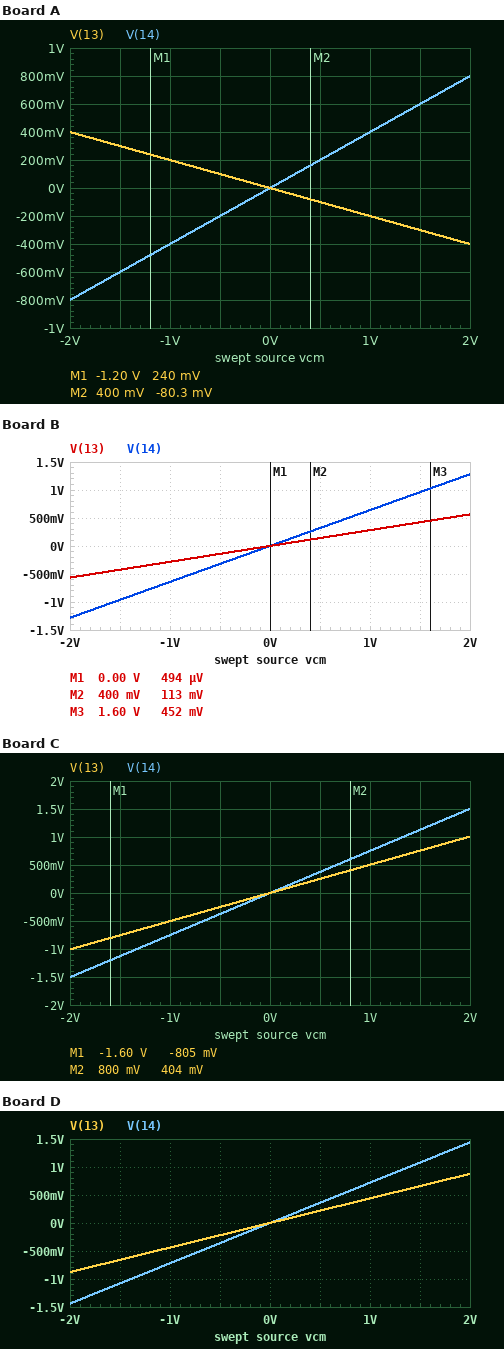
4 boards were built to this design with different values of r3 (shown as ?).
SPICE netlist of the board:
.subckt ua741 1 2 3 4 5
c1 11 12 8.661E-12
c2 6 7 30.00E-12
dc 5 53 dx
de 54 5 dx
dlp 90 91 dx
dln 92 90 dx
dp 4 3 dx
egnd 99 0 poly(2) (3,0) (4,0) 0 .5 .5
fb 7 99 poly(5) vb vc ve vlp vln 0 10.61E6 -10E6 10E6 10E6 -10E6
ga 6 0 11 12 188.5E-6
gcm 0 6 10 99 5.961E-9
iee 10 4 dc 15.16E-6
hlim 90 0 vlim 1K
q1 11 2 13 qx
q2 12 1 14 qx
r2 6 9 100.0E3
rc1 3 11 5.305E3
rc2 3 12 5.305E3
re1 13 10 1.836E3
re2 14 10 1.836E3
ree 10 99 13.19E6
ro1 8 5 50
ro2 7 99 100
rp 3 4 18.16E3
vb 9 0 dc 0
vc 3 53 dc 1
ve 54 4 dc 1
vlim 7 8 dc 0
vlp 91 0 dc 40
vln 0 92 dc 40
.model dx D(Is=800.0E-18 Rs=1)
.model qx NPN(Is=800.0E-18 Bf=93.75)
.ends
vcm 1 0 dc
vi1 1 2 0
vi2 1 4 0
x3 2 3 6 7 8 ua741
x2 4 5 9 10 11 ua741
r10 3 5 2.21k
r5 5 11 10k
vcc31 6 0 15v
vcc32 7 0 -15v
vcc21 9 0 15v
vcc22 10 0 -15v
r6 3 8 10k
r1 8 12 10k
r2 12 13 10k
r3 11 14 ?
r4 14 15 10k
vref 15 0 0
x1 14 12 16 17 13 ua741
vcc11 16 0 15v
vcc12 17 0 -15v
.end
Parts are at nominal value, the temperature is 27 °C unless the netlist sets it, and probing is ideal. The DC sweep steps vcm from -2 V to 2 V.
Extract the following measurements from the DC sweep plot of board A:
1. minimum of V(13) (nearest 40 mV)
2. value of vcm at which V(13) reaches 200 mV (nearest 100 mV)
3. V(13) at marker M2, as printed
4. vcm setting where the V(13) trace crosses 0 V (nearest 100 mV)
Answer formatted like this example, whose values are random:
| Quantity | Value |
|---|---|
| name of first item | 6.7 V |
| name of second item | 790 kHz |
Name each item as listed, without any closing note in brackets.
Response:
| Quantity | Value |
|---|---|
| minimum of V(13) | -400 mV |
| value of vcm at which V(13) reaches 200 mV | -1.0 V |
| V(13) at marker M2, as printed | -80.3 mV |
| vcm setting where the V(13) trace crosses 0 V | 0 V |
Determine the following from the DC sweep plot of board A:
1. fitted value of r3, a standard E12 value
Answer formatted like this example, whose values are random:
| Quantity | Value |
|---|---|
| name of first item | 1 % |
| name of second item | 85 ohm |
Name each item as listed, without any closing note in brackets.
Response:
| Quantity | Value |
|---|---|
| fitted value of r3, a standard E12 value | 15 kΩ |
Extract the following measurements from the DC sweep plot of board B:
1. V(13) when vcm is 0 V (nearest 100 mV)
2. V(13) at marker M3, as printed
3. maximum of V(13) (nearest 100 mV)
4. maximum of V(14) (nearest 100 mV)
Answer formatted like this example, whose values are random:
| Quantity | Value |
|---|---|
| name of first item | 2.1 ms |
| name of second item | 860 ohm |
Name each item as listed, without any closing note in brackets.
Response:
| Quantity | Value |
|---|---|
| V(13) when vcm is 0 V | 0 V |
| V(13) at marker M3, as printed | 452 mV |
| maximum of V(13) | 600 mV |
| maximum of V(14) | 1.3 V |
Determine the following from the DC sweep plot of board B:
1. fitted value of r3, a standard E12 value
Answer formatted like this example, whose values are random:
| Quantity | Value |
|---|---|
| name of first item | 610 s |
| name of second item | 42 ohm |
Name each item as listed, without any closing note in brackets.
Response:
| Quantity | Value |
|---|---|
| fitted value of r3, a standard E12 value | 5.6 kΩ |
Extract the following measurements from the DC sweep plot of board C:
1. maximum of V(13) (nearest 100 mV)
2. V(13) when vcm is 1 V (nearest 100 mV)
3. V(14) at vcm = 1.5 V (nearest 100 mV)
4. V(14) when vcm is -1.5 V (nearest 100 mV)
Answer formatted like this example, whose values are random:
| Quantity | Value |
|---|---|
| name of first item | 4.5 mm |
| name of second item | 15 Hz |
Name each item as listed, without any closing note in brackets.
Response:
| Quantity | Value |
|---|---|
| maximum of V(13) | 1.0 V |
| V(13) when vcm is 1 V | 500 mV |
| V(14) at vcm = 1.5 V | 1.1 V |
| V(14) when vcm is -1.5 V | -1.1 V |
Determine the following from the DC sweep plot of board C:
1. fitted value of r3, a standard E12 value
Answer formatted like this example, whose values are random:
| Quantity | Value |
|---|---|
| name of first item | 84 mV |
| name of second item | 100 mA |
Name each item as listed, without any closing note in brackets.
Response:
| Quantity | Value |
|---|---|
| fitted value of r3, a standard E12 value | 3.3 kΩ |
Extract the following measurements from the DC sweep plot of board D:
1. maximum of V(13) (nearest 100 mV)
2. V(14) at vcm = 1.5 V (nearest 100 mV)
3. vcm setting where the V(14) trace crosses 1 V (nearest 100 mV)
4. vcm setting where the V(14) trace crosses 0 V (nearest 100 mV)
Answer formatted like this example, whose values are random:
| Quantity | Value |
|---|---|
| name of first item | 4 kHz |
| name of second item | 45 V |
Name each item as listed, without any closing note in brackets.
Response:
| Quantity | Value |
|---|---|
| maximum of V(13) | 900 mV |
| V(14) at vcm = 1.5 V | 1.1 V |
| vcm setting where the V(14) trace crosses 1 V | 1.4 V |
| vcm setting where the V(14) trace crosses 0 V | 0 V |
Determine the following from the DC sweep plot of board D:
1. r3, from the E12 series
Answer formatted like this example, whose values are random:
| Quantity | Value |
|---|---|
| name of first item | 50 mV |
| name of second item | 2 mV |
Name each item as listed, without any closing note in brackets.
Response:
| Quantity | Value |
|---|---|
| r3, from the E12 series | 3.9 kΩ |
